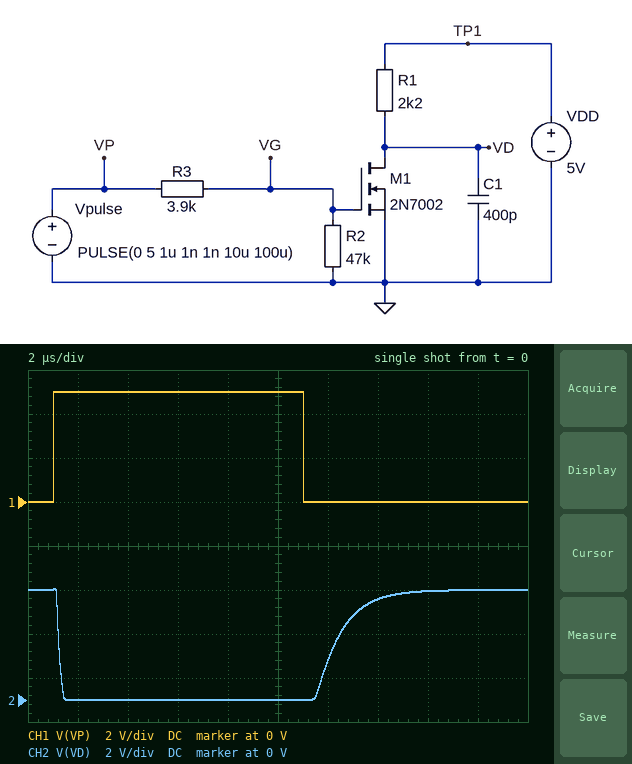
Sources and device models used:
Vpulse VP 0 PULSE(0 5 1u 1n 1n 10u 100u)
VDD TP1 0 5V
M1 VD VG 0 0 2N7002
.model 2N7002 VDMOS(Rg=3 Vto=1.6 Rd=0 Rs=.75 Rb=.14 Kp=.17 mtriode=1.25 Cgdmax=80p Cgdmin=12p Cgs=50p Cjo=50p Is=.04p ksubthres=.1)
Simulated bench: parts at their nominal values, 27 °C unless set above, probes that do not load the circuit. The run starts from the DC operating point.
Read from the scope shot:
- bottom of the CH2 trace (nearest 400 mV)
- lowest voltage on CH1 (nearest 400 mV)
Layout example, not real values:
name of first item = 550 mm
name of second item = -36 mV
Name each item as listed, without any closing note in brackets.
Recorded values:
bottom of the CH2 trace = 0 V
lowest voltage on CH1 = 0 V
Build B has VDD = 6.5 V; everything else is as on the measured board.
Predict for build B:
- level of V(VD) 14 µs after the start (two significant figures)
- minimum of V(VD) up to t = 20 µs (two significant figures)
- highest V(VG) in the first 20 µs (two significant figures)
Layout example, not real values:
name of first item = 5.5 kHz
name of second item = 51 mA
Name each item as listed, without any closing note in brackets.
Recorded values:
level of V(VD) 14 µs after the start = 6.0 V
minimum of V(VD) up to t = 20 µs = 4.7 mV
highest V(VG) in the first 20 µs = 4.6 V
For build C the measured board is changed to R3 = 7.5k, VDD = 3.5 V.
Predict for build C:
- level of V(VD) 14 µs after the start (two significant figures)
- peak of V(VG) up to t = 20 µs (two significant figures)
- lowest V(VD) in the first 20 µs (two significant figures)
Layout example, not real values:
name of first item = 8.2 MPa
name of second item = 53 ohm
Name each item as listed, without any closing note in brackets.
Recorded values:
level of V(VD) 14 µs after the start = 3.0 V
peak of V(VG) up to t = 20 µs = 4.3 V
lowest V(VD) in the first 20 µs = 2.8 mV
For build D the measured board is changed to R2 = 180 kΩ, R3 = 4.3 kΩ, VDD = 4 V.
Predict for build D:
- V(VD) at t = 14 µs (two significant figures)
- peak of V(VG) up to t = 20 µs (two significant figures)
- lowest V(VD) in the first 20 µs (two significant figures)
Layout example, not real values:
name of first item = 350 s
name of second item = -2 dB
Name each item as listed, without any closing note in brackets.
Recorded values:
V(VD) at t = 14 µs = 3.6 V
peak of V(VG) up to t = 20 µs = 4.9 V
lowest V(VD) in the first 20 µs = 2.1 mV
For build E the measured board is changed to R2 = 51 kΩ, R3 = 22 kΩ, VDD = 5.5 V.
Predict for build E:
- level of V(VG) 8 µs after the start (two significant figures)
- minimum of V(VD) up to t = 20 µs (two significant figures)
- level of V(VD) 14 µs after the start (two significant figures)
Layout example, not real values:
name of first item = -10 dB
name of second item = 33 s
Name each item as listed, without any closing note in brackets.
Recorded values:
level of V(VG) 8 µs after the start = 3.3 V
minimum of V(VD) up to t = 20 µs = 7.8 mV
level of V(VD) 14 µs after the start = 2.7 V
